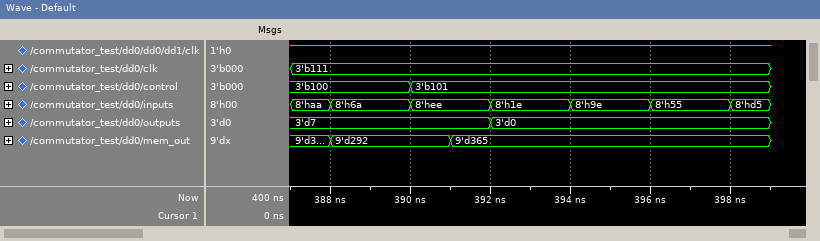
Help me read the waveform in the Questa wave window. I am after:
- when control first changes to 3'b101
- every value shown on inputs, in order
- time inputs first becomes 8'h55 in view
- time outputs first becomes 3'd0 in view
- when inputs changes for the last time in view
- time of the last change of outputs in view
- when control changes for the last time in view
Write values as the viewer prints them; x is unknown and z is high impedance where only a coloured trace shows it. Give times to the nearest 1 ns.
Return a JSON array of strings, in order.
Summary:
["390 ns", "8'haa, 8'h6a, 8'hee, 8'h1e, 8'h9e, 8'h55, 8'hd5", "396 ns", "392 ns", "398 ns", "392 ns", "390 ns"]
